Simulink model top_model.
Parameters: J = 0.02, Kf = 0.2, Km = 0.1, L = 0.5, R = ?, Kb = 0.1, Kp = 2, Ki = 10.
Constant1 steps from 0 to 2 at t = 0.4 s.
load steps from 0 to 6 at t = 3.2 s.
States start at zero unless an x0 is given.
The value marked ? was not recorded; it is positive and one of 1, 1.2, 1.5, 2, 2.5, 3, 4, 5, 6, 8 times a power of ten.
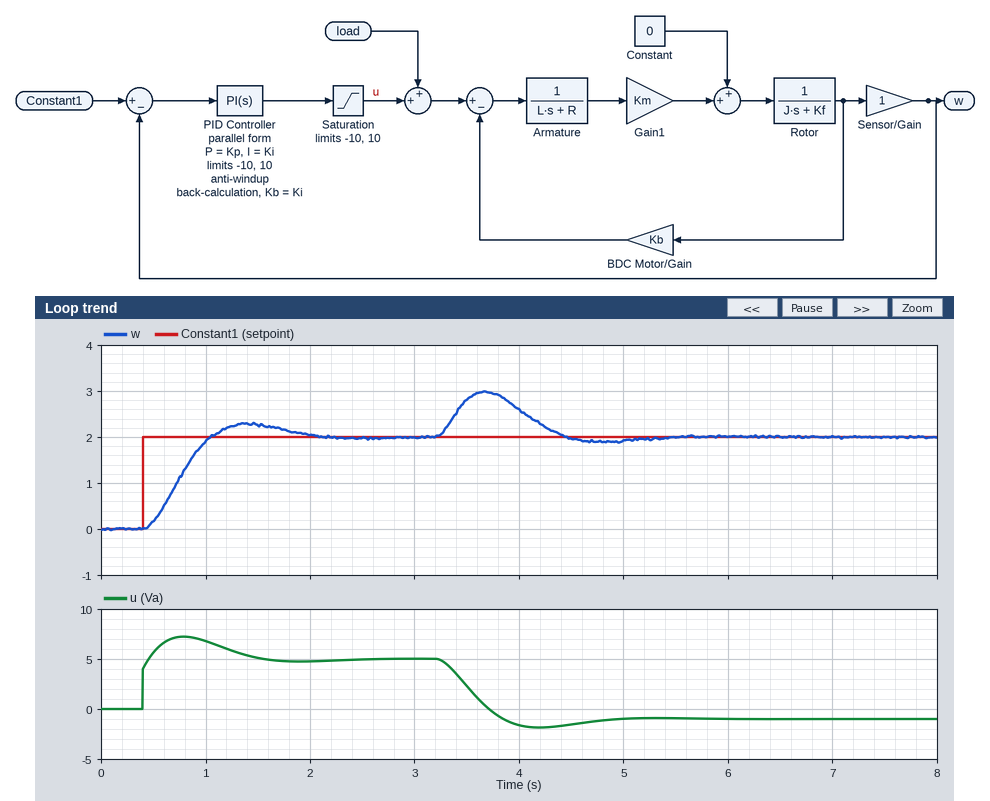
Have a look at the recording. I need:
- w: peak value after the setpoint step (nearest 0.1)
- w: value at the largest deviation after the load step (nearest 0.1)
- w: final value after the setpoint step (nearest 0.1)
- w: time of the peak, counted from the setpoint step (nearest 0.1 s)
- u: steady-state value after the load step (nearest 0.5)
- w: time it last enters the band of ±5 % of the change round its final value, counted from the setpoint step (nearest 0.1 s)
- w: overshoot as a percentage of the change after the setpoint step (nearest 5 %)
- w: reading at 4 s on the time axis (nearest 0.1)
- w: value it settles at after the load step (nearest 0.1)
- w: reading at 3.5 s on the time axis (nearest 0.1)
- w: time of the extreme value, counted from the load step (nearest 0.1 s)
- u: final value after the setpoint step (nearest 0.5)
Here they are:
2.3
3.0
2.0
1.0 s
-1.0
1.5 s
15 %
2.6
2.0
2.8
0.5 s
5.0
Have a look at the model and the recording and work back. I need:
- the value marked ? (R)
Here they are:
1.2
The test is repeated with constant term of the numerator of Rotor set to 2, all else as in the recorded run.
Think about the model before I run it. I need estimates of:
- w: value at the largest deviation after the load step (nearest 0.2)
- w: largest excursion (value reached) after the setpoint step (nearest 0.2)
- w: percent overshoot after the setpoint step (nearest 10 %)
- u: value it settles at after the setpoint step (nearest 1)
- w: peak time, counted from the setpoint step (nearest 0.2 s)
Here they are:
3.4
2.4
20 %
3
0.6 s
